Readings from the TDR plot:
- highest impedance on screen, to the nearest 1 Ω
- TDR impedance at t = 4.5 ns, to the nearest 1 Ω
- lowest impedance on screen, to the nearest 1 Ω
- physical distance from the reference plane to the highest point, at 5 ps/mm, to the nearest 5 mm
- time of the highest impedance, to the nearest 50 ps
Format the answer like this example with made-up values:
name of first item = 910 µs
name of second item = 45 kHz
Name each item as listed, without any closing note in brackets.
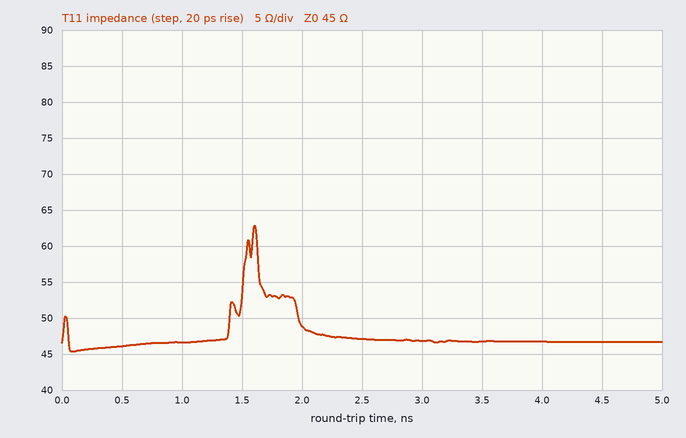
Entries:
highest impedance on screen, to the nearest 1 Ω = 63 Ω
TDR impedance at t = 4.5 ns, to the nearest 1 Ω = 47 Ω
lowest impedance on screen, to the nearest 1 Ω = 45 Ω
physical distance from the reference plane to the highest point, at 5 ps/mm, to the nearest 5 mm = 160 mm
time of the highest impedance, to the nearest 50 ps = 1.60 ns
